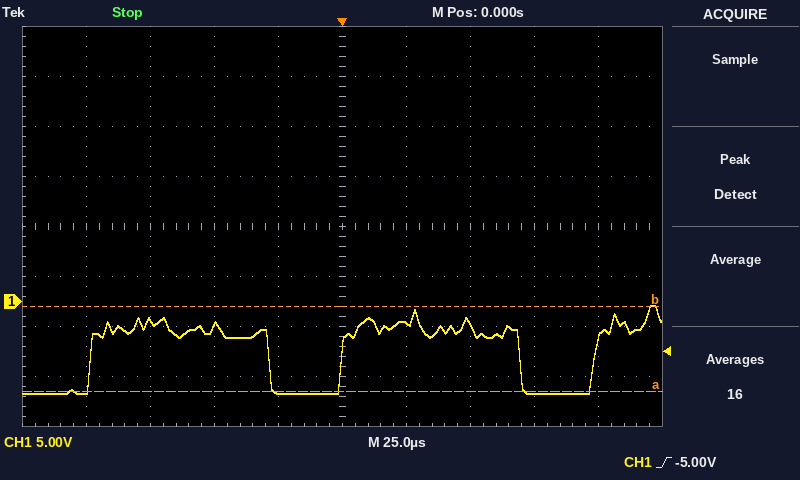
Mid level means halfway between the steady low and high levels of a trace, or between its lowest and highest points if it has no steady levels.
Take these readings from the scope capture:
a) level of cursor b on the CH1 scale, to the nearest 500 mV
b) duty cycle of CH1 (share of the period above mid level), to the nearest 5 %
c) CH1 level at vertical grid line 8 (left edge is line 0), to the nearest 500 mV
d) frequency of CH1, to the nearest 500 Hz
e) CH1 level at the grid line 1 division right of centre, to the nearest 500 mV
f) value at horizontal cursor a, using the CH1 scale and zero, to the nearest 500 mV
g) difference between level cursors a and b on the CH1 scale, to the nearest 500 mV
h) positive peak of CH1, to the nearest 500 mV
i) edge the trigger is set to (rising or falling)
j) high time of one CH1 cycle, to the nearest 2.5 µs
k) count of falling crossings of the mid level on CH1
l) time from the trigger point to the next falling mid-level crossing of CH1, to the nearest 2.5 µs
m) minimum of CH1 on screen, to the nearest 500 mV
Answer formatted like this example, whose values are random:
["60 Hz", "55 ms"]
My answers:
["-500 mV", "70 %", "-9.0 V", "10.0 kHz", "-2.0 V", "-9.0 V", "8.5 V", "-500 mV", "rising", "70.0 µs", "2", "70.0 µs", "-9.0 V"]
